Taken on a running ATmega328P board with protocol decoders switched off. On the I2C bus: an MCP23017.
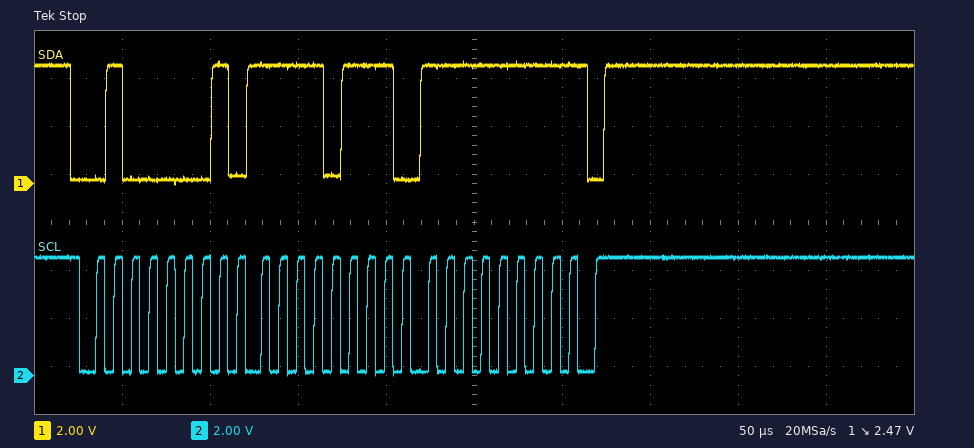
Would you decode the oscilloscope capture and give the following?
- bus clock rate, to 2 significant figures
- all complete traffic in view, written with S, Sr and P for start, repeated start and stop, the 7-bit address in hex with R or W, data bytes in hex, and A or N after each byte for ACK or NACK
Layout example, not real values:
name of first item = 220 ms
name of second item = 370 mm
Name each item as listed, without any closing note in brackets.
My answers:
bus clock rate, to 2 significant figures = 100 kHz
all complete traffic in view, written with S, Sr and P for start, repeated start and stop, the 7-bit address in hex with R or W, data bytes in hex, and A or N after each byte for ACK or NACK = S 20R A F7 A FF N P
